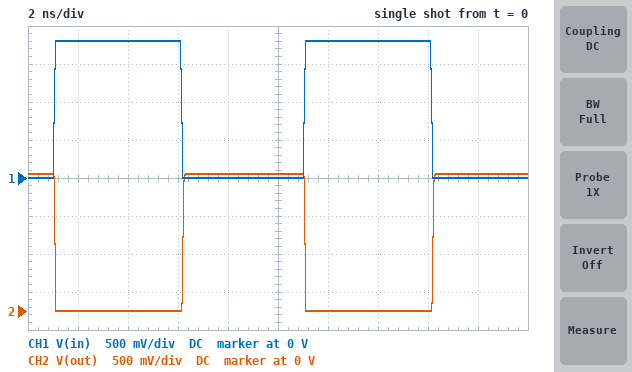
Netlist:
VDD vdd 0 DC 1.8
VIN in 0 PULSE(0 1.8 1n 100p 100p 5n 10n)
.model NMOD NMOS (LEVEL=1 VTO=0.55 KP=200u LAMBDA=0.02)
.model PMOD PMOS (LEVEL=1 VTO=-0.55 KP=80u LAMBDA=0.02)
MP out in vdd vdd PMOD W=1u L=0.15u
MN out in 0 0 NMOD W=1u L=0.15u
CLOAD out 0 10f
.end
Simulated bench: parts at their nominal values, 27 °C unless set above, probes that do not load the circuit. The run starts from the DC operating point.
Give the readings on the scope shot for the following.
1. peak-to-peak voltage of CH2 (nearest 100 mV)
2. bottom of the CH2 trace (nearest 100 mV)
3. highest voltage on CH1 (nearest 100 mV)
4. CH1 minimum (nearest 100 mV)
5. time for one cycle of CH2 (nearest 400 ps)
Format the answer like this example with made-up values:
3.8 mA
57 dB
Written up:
1.8 V
0 V
1.8 V
0 V
10.0 ns
